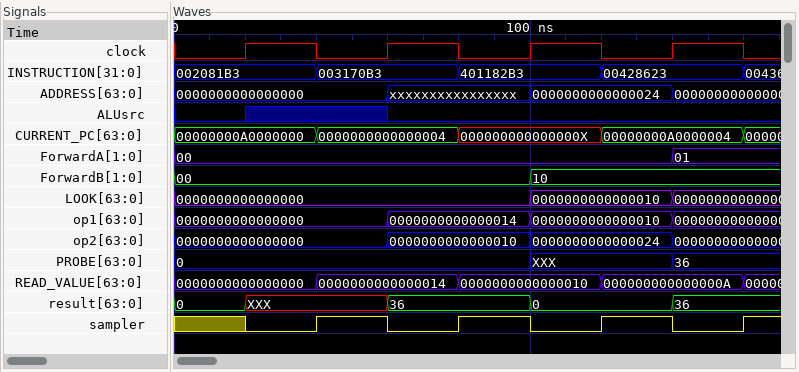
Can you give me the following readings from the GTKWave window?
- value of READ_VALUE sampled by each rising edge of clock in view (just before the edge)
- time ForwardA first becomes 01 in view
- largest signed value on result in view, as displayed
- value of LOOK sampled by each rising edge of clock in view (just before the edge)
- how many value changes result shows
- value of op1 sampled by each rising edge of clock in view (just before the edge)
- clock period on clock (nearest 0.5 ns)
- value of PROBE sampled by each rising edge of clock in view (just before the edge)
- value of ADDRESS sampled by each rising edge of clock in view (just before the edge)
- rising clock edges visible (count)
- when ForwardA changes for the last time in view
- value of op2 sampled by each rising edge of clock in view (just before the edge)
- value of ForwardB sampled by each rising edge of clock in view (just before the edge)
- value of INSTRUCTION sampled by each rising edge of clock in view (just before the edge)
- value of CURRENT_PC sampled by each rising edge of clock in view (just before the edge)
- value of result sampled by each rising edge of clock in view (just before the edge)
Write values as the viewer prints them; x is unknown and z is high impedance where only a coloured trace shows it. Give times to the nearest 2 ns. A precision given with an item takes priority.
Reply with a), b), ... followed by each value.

a) 0000000000000000, 0000000000000014, 0000000000000010, 000000000000000A
b) 140 ns
c) 36
d) 0000000000000000, 0000000000000000, 0000000000000000, 0000000000000010
e) 4
f) 0000000000000000, 0000000000000000, 0000000000000014, 0000000000000010
g) 40 ns
h) 0, 0, 0, XXX
i) 0000000000000000, 0000000000000000, xxxxxxxxxxxxxxxx, 0000000000000024
j) 4
k) 140 ns
l) 0000000000000000, 0000000000000000, 0000000000000010, 0000000000000024
m) 00, 00, 00, 10
n) 002081B3, 003170B3, 401182B3, 00428623
o) 00000000A0000000, 0000000000000004, 000000000000000X, 00000000A0000004
p) 0, XXX, 36, 0
